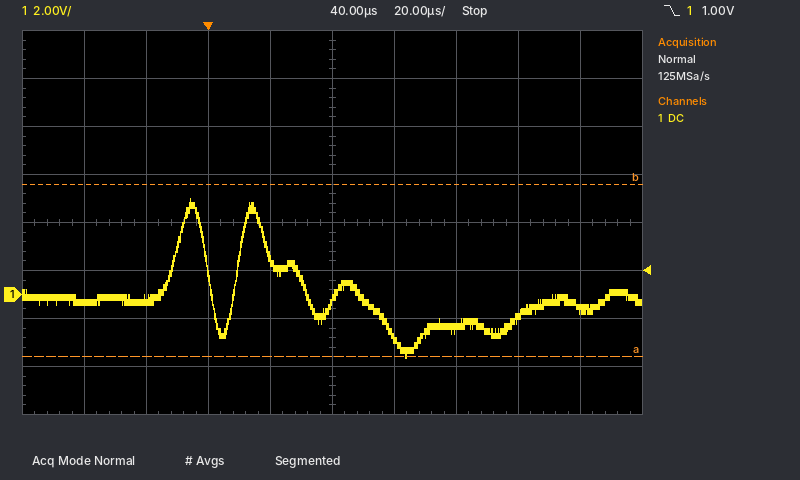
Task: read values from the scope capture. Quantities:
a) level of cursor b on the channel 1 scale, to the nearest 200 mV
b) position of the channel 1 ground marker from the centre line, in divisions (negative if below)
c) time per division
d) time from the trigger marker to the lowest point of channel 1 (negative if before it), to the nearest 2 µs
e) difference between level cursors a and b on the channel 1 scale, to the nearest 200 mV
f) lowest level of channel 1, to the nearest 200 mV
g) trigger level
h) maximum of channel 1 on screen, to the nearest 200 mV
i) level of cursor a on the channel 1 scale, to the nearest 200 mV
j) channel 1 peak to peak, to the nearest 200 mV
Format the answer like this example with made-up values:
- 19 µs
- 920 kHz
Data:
- 4.6 V
- -1.5 div
- 20 µs
- +64 µs
- 7.2 V
- -2.6 V
- 1.00 V
- 4.0 V
- -2.6 V
- 6.6 V
